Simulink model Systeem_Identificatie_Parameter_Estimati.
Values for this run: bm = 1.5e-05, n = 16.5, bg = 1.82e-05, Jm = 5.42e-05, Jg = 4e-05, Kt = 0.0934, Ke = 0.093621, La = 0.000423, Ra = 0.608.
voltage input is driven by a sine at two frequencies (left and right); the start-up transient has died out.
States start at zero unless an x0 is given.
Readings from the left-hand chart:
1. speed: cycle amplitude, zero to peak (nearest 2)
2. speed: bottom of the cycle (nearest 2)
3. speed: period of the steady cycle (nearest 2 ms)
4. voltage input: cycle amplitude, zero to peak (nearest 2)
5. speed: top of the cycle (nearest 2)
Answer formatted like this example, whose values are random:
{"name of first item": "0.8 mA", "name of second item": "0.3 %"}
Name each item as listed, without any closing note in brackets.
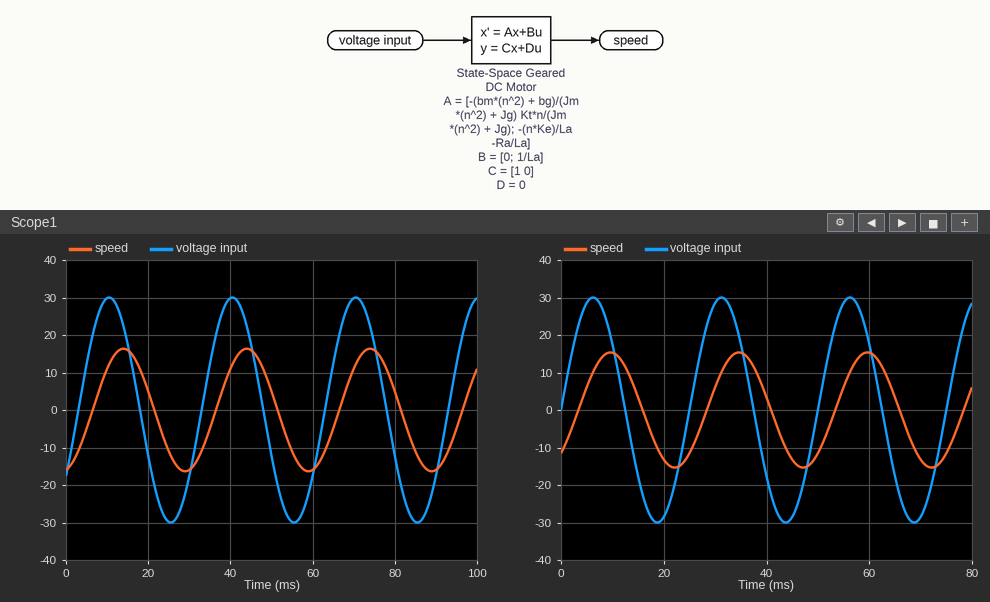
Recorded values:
{"speed: cycle amplitude, zero to peak": "16", "speed: bottom of the cycle": "-16", "speed: period of the steady cycle": "30 ms", "voltage input: cycle amplitude, zero to peak": "30", "speed: top of the cycle": "16"}
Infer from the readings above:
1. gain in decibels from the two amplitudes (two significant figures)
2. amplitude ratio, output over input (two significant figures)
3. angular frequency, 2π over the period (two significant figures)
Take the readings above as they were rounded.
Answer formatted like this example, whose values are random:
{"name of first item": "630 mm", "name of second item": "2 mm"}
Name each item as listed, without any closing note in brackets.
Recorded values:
{"gain in decibels from the two amplitudes": "-5.5 dB", "amplitude ratio, output over input": "0.53", "angular frequency, 2π over the period": "0.21 rad/ms"}
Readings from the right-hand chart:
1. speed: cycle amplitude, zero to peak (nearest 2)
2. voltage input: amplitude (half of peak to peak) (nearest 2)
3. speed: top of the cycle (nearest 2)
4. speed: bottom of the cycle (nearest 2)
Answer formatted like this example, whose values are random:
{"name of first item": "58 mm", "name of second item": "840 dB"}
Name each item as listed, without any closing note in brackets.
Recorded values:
{"speed: cycle amplitude, zero to peak": "16", "voltage input: amplitude (half of peak to peak)": "30", "speed: top of the cycle": "16", "speed: bottom of the cycle": "-16"}
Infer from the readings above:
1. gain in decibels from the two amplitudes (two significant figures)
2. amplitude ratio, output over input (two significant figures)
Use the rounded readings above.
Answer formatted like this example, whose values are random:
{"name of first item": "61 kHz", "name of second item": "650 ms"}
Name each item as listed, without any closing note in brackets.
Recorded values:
{"gain in decibels from the two amplitudes": "-5.5 dB", "amplitude ratio, output over input": "0.53"}
